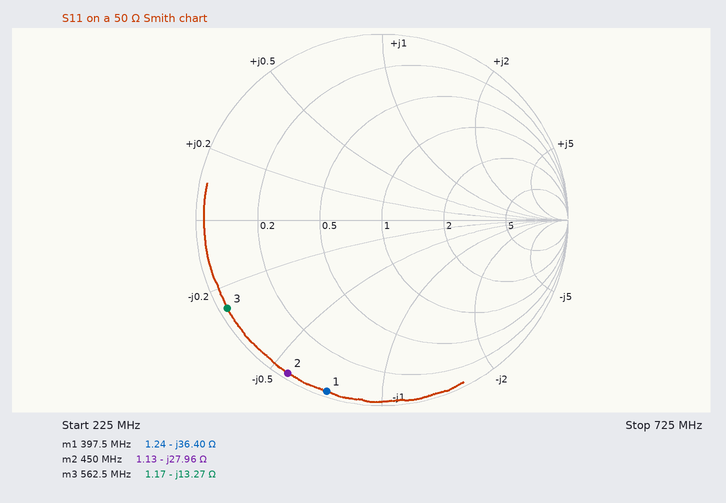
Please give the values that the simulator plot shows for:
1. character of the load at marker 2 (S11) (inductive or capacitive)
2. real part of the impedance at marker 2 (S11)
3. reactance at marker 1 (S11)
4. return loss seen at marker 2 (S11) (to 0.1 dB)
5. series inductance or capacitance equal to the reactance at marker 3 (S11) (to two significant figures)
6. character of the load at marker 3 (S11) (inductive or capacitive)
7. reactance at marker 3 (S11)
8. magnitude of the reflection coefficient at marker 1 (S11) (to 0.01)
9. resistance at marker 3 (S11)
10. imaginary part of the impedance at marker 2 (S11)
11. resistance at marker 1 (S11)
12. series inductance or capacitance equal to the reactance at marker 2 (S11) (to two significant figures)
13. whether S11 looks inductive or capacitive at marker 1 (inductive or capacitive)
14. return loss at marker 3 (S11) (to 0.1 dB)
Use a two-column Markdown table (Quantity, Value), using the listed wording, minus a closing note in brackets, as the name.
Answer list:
| Quantity | Value |
|---|---|
| character of the load at marker 2 (S11) | capacitive |
| real part of the impedance at marker 2 | 1.13 Ω |
| reactance at marker 1 | -36.40 Ω |
| return loss seen at marker 2 (S11) | 0.3 dB |
| series inductance or capacitance equal to the reactance at marker 3 (S11) | 21 pF |
| character of the load at marker 3 (S11) | capacitive |
| reactance at marker 3 | -13.27 Ω |
| magnitude of the reflection coefficient at marker 1 (S11) | 0.97 |
| resistance at marker 3 | 1.17 Ω |
| imaginary part of the impedance at marker 2 | -27.96 Ω |
| resistance at marker 1 | 1.24 Ω |
| series inductance or capacitance equal to the reactance at marker 2 (S11) | 13 pF |
| whether S11 looks inductive or capacitive at marker 1 | capacitive |
| return loss at marker 3 (S11) | 0.4 dB |
